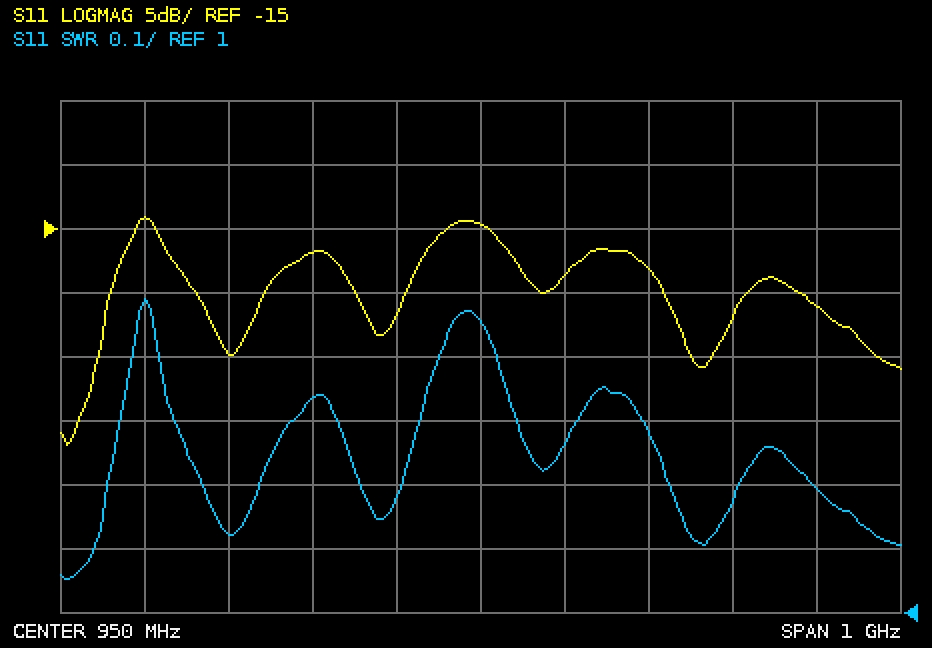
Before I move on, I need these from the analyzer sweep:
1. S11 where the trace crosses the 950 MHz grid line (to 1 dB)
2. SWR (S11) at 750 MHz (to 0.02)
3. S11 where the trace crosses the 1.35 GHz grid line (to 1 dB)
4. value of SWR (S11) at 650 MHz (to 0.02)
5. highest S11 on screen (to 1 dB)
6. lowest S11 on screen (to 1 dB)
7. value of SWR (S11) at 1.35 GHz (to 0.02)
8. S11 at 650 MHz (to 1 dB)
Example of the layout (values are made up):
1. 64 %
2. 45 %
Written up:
1. -15 dB
2. 1.34
3. -21 dB
4. 1.12
5. -14 dB
6. -32 dB
7. 1.20
8. -25 dB
